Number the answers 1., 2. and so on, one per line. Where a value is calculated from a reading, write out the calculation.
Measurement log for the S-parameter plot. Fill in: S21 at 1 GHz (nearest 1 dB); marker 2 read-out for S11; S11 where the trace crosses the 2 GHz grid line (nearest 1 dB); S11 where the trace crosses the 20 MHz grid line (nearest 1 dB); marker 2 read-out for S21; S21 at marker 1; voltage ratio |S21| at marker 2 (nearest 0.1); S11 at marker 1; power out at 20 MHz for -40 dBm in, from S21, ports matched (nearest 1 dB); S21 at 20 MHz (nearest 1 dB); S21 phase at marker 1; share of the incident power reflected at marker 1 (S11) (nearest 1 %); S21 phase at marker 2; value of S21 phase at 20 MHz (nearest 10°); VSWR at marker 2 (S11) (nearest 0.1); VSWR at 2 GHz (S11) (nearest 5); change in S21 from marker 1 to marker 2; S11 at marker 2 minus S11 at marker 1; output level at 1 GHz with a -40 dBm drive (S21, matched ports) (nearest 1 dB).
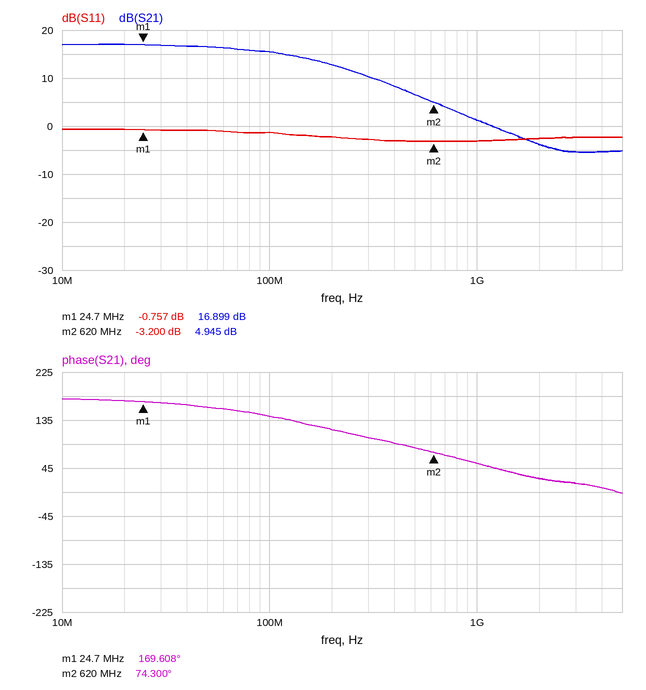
1. 1 dB
2. -3.200 dB
3. -3 dB
4. -1 dB
5. 4.945 dB
6. 16.899 dB
7. 10^(4.945/20) ≈ 1.8
8. -0.757 dB
9. -40 dBm + (17 dB) = -23 dBm
10. 17 dB
11. 169.608°
12. 10^(-0.757/10) ≈ 84 %
13. 74.300°
14. 170°
15. (1 + 0.6918)/(1 − 0.6918) ≈ 5.5
16. |Γ| = 10^(-3/20) = 0.7079; VSWR = (1 + 0.7079)/(1 − 0.7079) ≈ 5.85, so 5 to the nearest 5
17. 4.945 − (16.899) = -11.954 dB
18. -3.2 − (-0.757) = -2.443 dB
19. -40 dBm + (1 dB) = -39 dBm
